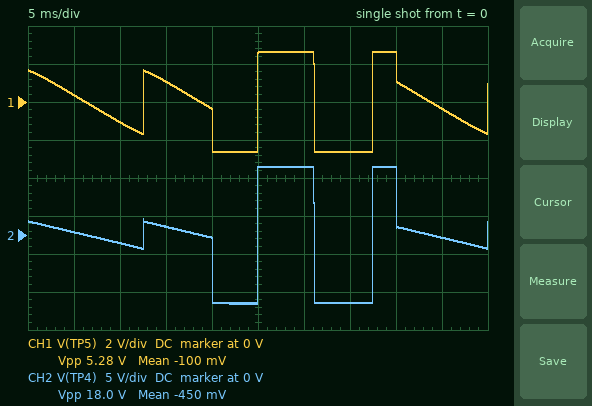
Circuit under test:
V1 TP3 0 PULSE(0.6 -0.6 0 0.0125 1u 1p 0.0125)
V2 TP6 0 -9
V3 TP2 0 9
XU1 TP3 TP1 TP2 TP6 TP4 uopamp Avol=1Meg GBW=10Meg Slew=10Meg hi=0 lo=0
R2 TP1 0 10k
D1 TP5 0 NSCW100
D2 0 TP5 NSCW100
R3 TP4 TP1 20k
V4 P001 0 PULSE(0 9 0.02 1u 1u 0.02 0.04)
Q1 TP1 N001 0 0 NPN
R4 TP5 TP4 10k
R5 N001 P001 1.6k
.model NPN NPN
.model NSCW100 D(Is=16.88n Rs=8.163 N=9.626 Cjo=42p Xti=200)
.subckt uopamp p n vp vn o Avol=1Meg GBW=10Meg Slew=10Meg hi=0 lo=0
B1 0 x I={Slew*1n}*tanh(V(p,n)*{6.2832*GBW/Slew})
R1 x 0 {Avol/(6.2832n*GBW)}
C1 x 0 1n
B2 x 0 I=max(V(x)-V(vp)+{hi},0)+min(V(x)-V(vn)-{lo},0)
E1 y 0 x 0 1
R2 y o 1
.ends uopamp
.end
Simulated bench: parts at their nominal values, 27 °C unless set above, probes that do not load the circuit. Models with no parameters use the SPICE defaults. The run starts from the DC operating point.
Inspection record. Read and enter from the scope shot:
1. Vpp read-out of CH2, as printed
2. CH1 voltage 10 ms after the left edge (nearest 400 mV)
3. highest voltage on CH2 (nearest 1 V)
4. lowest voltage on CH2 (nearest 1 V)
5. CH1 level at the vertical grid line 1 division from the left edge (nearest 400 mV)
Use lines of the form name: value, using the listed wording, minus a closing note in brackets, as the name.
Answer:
Vpp read-out of CH2, as printed: 18.0 V
CH1 voltage 10 ms after the left edge: -1.2 V
highest voltage on CH2: 9 V
lowest voltage on CH2: -9 V
CH1 level at the vertical grid line 1 division from the left edge: 400 mV
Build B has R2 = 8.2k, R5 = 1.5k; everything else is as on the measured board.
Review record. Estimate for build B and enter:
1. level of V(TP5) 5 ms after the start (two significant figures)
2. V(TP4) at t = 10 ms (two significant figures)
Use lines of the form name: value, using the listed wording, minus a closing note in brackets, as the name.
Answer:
level of V(TP5) 5 ms after the start: 410 mV
V(TP4) at t = 10 ms: -1.2 V
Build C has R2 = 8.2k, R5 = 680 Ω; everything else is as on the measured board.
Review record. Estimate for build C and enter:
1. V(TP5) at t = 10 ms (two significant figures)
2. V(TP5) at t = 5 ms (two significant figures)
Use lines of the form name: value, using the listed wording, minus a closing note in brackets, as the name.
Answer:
V(TP5) at t = 10 ms: -1.2 V
V(TP5) at t = 5 ms: 410 mV
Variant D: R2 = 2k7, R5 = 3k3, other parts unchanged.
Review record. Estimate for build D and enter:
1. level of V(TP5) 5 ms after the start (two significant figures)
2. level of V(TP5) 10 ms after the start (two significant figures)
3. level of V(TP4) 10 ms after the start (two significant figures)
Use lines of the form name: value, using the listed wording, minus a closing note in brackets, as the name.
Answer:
level of V(TP5) 5 ms after the start: 1.0 V
level of V(TP5) 10 ms after the start: -2.1 V
level of V(TP4) 10 ms after the start: -3.0 V
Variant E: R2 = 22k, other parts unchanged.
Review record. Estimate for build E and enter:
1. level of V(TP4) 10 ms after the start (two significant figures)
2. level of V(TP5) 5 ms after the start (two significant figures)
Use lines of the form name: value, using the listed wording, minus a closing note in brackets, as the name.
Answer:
level of V(TP4) 10 ms after the start: -690 mV
level of V(TP5) 5 ms after the start: 230 mV
